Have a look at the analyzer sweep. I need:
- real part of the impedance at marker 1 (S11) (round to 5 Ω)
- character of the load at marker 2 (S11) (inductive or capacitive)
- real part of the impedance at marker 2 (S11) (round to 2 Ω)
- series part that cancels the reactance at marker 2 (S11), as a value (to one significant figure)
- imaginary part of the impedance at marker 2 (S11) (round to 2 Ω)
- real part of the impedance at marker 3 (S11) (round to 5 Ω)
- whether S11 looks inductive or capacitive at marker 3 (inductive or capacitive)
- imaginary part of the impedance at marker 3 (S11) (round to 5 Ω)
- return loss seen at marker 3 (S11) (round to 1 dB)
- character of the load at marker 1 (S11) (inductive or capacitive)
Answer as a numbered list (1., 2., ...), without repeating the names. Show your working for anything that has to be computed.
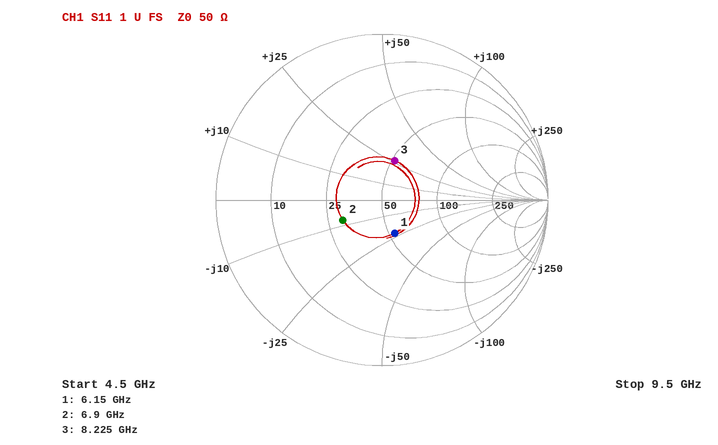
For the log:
1. 55 Ω
2. capacitive
3. 30 Ω
4. L = 8 Ω/(2π × 6.9 GHz) ≈ 185 pH, so 200 pH to one significant figure
5. -8 Ω
6. 50 Ω
7. inductive
8. +25 Ω
9. 12 dB
10. capacitive
